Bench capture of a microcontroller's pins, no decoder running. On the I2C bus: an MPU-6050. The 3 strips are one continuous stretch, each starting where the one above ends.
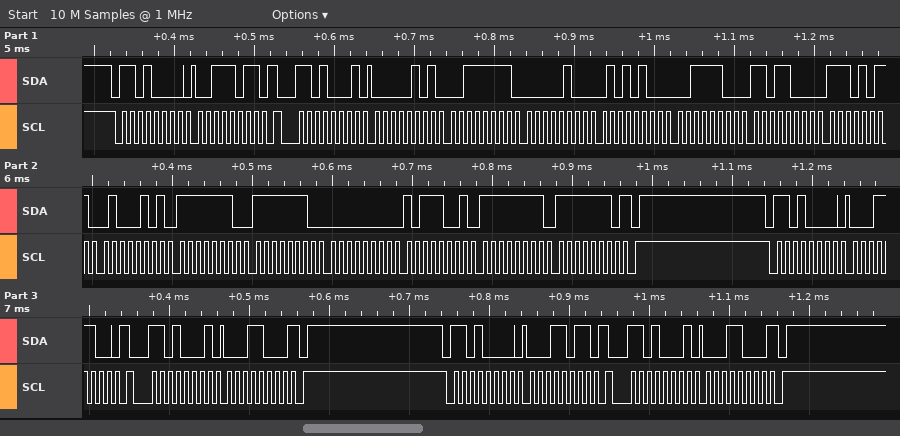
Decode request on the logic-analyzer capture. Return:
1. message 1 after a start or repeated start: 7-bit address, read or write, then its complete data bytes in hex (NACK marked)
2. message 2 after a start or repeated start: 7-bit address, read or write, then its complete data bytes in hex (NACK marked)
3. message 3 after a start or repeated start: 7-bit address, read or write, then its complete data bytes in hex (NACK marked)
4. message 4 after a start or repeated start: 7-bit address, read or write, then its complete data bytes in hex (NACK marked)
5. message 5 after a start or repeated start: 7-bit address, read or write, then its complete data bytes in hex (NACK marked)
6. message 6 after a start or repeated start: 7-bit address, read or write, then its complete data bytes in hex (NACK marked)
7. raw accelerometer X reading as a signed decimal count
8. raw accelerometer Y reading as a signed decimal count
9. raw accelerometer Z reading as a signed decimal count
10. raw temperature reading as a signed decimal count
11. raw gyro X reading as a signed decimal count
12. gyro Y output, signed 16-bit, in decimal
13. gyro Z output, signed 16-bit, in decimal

0x68 write: 3B
0x68 read: 05 3F 04 54 3C D8 EB 45 FE FE 00 B9 FF FE NACK
0x68 write: 1C
0x68 read: 18 NACK
0x68 write: 1B
0x68 read: 18 NACK
1343
1108
15576
-5307
-258
185
-2
